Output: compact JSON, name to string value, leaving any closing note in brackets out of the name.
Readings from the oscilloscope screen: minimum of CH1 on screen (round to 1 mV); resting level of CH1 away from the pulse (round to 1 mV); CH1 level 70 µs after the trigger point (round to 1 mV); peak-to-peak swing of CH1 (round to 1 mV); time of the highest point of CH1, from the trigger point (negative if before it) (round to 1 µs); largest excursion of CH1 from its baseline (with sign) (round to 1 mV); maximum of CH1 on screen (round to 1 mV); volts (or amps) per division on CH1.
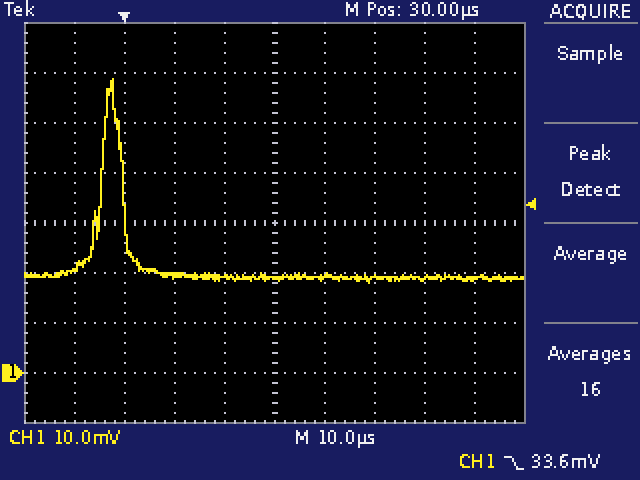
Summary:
{"minimum of CH1 on screen": "18 mV", "resting level of CH1 away from the pulse": "19 mV", "CH1 level 70 µs after the trigger point": "19 mV", "peak-to-peak swing of CH1": "41 mV", "time of the highest point of CH1, from the trigger point (negative if before it)": "-2 µs", "largest excursion of CH1 from its baseline (with sign)": "+40 mV", "maximum of CH1 on screen": "59 mV", "volts (or amps) per division on CH1": "10 mV"}
